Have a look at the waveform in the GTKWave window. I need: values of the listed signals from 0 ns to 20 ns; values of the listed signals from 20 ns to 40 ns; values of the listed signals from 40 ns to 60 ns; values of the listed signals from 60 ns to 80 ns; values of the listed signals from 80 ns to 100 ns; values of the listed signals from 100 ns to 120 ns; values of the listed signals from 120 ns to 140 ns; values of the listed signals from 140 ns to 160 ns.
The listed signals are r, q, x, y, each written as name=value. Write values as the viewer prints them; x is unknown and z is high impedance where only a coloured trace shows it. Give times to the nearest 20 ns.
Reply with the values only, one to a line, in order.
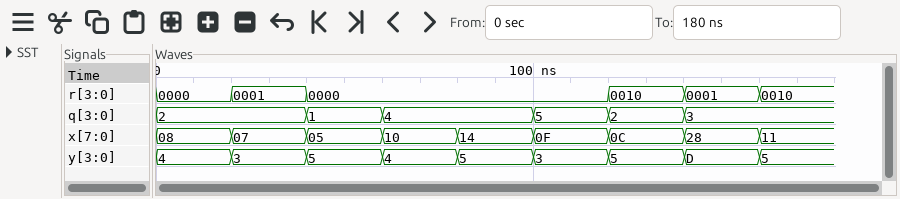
r=0000, q=2, x=08, y=4
r=0001, q=2, x=07, y=3
r=0000, q=1, x=05, y=5
r=0000, q=4, x=10, y=4
r=0000, q=4, x=14, y=5
r=0000, q=5, x=0F, y=3
r=0010, q=2, x=0C, y=5
r=0001, q=3, x=28, y=D
